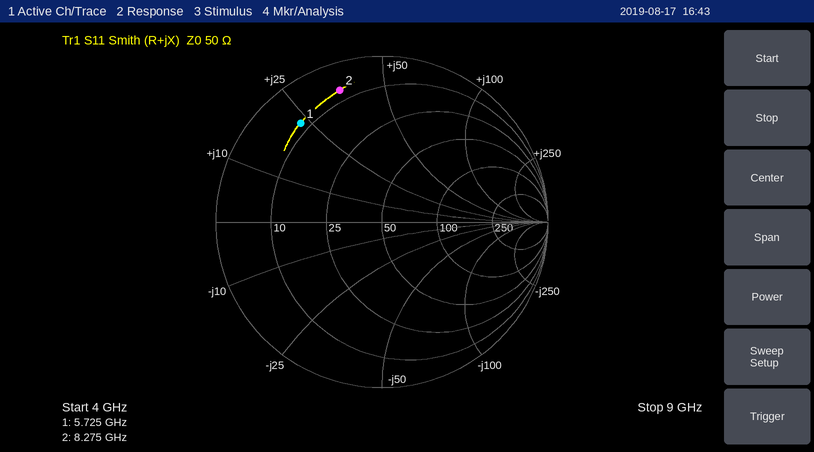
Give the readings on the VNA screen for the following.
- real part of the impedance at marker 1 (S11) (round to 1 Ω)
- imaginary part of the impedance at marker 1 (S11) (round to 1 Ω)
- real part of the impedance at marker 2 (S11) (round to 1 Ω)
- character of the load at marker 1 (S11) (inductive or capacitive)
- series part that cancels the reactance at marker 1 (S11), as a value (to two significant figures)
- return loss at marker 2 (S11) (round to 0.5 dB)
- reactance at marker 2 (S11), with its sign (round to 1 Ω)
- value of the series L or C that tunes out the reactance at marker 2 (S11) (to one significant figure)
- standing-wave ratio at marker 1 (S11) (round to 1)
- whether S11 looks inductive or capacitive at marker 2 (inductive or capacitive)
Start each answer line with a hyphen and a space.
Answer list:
- 8 Ω
- +23 Ω
- 7 Ω
- inductive
- 1.2 pF
- 1.5 dB
- +36 Ω
- 500 fF
- 8
- inductive
